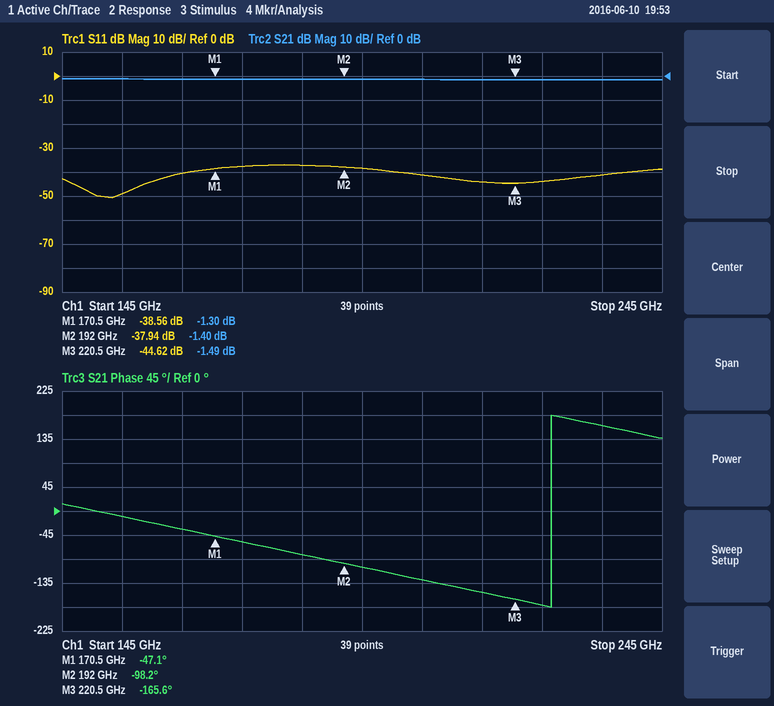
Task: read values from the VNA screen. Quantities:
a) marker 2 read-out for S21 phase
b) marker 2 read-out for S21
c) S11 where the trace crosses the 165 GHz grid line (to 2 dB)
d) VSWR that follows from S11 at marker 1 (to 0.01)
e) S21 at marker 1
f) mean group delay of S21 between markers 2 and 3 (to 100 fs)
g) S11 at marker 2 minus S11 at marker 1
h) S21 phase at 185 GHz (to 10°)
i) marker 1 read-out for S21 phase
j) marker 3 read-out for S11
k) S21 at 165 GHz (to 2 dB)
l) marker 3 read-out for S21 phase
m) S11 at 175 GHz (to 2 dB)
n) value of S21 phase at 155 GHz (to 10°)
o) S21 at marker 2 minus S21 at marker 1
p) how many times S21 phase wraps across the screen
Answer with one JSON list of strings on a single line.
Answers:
["-98.2°", "-1.40 dB", "-40 dB", "1.02", "-1.30 dB", "6.6 ps", "0.62 dB", "-80°", "-47.1°", "-44.62 dB", "-2 dB", "-165.6°", "-38 dB", "-10°", "-0.10 dB", "1"]
